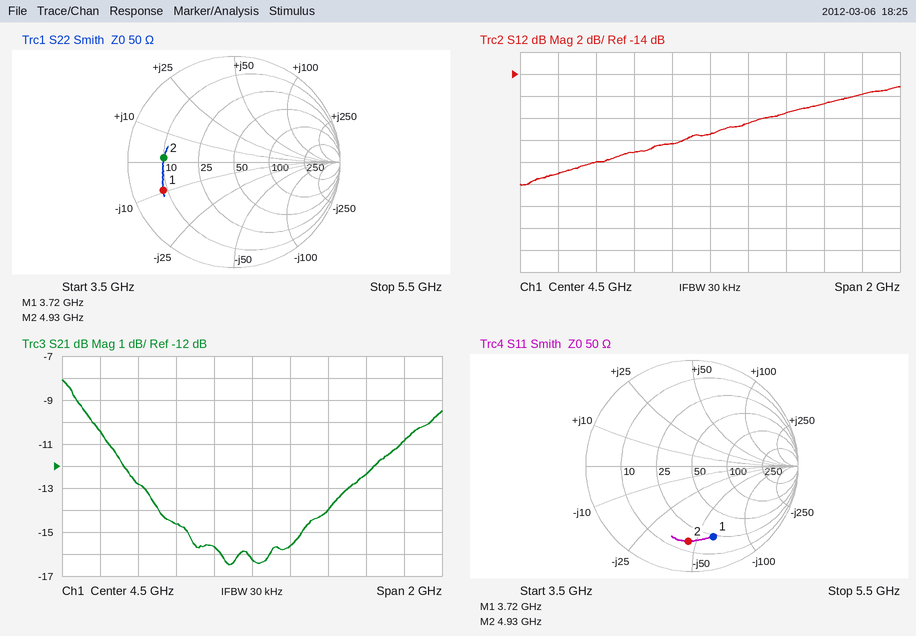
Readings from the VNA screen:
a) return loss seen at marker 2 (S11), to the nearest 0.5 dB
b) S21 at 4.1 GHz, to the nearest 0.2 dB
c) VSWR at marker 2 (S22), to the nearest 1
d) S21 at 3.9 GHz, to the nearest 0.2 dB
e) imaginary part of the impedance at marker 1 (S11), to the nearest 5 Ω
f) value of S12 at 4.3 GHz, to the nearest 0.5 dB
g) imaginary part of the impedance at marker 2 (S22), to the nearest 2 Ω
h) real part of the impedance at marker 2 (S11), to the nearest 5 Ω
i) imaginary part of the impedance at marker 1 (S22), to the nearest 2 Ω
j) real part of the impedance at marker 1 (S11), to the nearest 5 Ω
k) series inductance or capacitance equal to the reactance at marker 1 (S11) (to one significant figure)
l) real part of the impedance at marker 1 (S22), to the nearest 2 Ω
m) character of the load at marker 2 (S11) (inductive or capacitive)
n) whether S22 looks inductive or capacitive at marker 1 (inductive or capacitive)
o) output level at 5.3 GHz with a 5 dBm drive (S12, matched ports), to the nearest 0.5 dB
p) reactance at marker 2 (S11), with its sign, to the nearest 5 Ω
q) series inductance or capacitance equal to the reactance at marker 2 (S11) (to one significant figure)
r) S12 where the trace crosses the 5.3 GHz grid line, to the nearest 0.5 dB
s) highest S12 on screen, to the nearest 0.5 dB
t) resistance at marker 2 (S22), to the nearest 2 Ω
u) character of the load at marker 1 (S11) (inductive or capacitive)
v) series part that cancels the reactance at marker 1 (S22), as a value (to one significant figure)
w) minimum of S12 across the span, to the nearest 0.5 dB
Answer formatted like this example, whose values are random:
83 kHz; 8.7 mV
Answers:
3.0 dB; -14.6 dB; 5; -12.8 dB; -60 Ω; -20.5 dB; +2 Ω; 15 Ω; -10 Ω; 25 Ω; 700 fF; 8 Ω; capacitive; capacitive; -11.0 dBm; -45 Ω; 700 fF; -16.0 dB; -15.0 dB; 10 Ω; capacitive; 400 pH; -24.0 dB
